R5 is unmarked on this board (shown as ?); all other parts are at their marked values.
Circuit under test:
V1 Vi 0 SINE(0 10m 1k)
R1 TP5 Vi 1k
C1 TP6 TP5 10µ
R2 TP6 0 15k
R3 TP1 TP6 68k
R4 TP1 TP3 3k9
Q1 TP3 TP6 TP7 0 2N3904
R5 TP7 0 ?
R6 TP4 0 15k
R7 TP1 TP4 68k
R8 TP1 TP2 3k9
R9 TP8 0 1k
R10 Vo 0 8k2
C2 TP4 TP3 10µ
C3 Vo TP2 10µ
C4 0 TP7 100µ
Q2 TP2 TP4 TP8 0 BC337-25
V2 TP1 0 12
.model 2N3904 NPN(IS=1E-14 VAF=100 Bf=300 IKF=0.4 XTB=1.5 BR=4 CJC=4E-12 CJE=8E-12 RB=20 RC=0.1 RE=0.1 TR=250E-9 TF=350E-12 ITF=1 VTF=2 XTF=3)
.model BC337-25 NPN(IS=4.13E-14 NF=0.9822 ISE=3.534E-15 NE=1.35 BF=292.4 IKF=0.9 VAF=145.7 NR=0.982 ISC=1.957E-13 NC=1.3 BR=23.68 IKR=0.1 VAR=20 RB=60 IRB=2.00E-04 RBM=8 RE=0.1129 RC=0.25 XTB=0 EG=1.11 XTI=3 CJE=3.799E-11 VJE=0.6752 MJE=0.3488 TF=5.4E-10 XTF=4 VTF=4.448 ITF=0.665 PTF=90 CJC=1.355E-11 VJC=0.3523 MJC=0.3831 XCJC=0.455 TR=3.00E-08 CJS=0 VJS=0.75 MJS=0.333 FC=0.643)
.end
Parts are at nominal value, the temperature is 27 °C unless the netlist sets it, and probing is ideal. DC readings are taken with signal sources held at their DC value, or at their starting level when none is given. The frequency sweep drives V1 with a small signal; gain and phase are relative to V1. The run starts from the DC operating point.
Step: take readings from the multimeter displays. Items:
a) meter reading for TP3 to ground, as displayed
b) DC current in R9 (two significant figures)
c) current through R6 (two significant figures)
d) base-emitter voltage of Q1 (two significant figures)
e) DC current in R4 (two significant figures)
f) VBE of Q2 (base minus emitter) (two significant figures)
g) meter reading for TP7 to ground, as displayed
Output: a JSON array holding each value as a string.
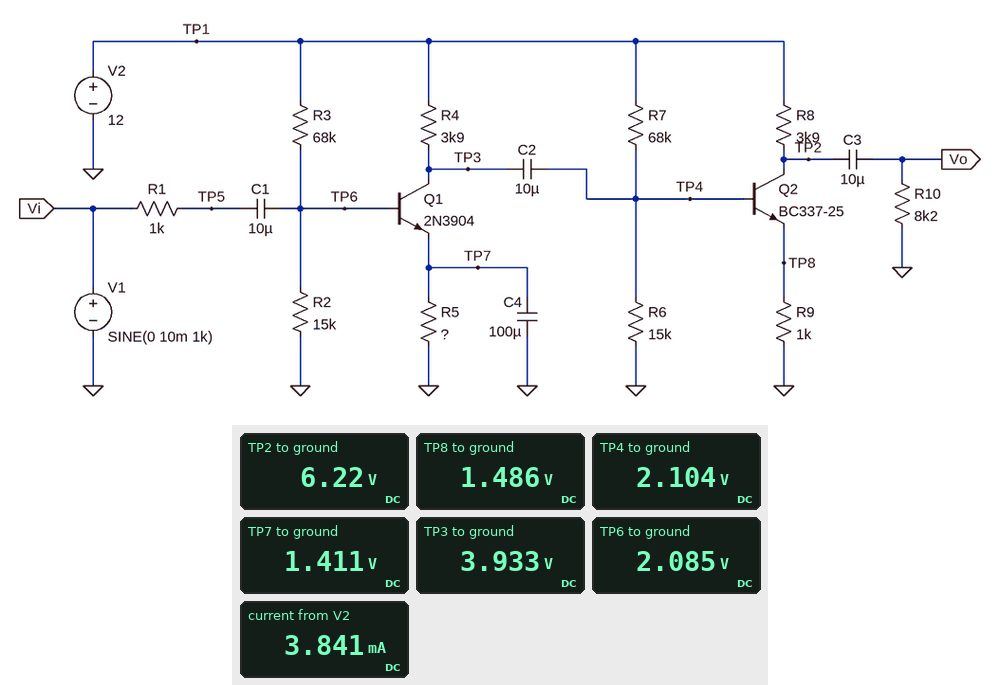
["3.933 V", "1.5 mA", "140 µA", "670 mV", "2.1 mA", "620 mV", "1.411 V"]
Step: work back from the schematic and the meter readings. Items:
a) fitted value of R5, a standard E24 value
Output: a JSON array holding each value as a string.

["680 Ω"]
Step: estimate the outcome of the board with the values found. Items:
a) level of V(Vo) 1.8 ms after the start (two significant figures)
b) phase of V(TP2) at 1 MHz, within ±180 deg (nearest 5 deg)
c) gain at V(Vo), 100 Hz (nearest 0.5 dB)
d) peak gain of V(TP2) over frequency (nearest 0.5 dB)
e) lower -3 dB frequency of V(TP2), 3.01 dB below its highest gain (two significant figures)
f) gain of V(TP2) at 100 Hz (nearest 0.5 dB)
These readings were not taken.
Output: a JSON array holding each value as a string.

["-3.4 V", "-80 deg", "49.5 dB", "52.5 dB", "100 Hz", "49.5 dB"]
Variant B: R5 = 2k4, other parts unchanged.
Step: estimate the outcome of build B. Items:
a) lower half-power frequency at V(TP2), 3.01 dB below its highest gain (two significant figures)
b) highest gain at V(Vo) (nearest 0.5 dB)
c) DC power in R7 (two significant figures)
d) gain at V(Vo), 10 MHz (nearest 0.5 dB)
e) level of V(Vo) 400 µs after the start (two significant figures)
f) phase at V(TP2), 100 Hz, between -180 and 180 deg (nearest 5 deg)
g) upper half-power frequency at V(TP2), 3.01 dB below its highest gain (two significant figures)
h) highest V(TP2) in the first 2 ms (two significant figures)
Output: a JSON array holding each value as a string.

["37 Hz", "44.0 dB", "1.4 mW", "20.0 dB", "850 mV", "20 deg", "830 kHz", "7.9 V"]
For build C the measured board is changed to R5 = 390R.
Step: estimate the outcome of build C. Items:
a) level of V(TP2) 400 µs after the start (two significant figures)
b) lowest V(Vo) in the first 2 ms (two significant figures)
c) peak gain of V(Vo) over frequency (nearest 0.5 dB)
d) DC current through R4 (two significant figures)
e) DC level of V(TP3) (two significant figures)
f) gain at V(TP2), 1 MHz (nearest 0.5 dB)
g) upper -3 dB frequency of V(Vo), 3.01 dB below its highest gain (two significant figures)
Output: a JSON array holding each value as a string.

["6.2 V", "-35 mV", "8.5 dB", "2.8 mA", "1.2 V", "-7.0 dB", "170 kHz"]
